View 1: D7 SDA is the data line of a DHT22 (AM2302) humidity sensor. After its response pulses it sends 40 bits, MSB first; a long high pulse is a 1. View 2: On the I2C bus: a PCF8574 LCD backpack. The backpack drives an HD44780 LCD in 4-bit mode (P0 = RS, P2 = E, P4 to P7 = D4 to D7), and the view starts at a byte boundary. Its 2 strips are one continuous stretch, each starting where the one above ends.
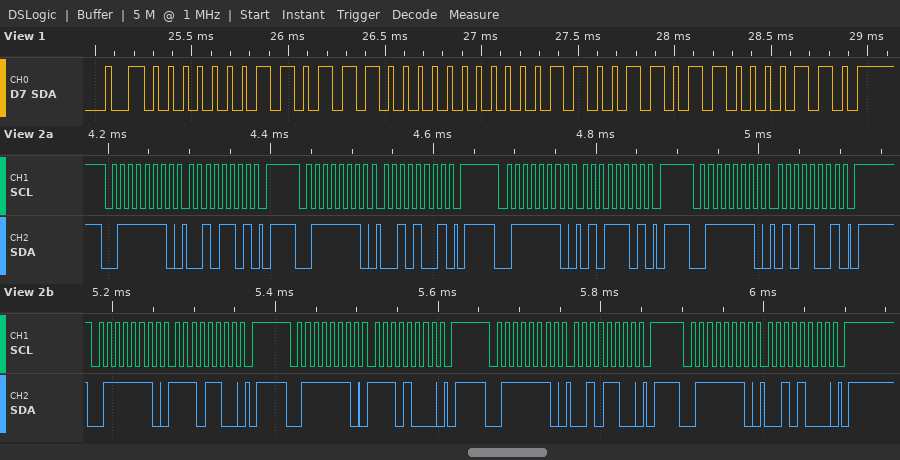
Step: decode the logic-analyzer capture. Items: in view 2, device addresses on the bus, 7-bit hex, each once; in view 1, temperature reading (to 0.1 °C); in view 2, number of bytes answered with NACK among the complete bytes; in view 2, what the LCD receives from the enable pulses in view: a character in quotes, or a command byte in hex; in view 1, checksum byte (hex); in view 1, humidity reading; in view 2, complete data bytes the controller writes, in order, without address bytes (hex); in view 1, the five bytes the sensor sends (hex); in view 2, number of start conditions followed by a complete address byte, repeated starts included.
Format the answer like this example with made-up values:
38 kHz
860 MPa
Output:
0x3F
20.5 °C
0
'%' 0xE2
0x86
44.0 %
2D 29 5D 59 EC E8 2C 28
01 B8 00 CD 86
8
